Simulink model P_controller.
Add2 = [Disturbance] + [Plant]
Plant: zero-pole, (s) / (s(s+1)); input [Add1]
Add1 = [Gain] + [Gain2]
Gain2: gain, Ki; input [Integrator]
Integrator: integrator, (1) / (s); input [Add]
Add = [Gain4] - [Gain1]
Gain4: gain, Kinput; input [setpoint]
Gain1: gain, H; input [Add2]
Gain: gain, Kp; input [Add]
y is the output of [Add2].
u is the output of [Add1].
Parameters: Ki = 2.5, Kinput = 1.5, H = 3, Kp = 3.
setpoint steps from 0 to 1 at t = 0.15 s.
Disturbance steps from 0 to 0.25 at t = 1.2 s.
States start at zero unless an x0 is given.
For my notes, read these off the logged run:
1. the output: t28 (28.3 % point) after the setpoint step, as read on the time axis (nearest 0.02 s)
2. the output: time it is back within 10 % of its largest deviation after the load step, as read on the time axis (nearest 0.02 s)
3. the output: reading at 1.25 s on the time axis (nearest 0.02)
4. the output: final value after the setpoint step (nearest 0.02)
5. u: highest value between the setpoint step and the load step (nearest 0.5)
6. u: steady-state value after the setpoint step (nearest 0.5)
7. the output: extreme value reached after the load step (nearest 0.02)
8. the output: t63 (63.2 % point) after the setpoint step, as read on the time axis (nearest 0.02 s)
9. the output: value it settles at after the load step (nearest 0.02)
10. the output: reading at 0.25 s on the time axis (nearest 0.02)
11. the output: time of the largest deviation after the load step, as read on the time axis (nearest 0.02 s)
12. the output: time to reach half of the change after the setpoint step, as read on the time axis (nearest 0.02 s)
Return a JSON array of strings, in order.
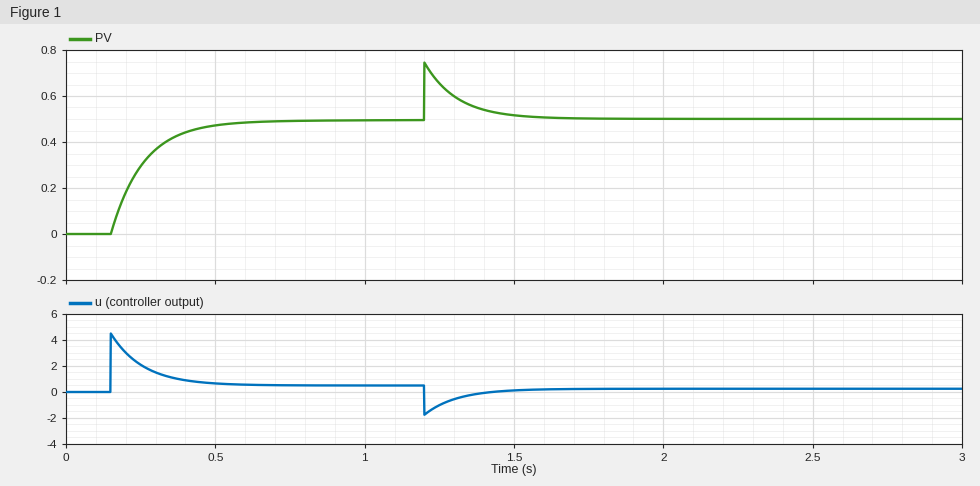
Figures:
["0.18 s", "1.46 s", "0.66", "0.50", "4.5", "0.5", "0.74", "0.26 s", "0.50", "0.30", "1.20 s", "0.22 s"]
